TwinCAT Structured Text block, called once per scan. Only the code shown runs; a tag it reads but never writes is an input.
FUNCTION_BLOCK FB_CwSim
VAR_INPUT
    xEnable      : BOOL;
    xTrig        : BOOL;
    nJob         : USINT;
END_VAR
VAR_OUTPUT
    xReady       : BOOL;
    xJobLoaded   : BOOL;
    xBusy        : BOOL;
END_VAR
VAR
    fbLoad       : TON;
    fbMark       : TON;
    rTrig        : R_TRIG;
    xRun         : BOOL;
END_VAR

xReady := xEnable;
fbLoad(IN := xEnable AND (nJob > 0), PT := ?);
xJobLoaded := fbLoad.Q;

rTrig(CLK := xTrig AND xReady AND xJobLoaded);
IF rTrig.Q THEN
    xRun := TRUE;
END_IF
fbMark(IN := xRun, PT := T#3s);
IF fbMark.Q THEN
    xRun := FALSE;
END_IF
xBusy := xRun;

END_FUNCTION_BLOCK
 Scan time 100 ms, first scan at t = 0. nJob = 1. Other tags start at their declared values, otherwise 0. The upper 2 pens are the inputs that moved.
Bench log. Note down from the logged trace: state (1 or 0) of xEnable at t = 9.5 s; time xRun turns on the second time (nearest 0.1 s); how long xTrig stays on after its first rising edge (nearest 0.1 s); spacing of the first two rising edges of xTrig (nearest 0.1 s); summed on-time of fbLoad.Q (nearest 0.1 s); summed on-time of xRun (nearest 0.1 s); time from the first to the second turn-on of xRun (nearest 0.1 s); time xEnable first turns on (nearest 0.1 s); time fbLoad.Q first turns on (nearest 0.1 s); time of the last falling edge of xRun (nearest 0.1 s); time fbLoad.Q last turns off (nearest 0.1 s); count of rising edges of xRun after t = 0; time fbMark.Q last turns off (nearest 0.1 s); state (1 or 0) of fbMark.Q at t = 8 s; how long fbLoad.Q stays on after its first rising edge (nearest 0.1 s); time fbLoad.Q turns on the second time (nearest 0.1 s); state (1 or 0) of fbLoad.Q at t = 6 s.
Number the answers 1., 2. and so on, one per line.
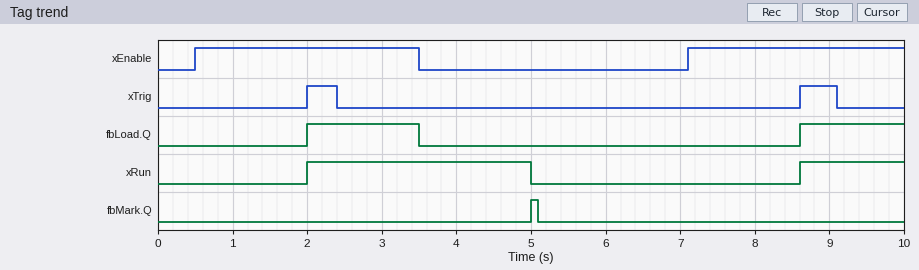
1. 1
2. 8.6 s
3. 0.4 s
4. 6.6 s
5. 2.9 s
6. 4.4 s
7. 6.6 s
8. 0.5 s
9. 2.0 s
10. 5.0 s
11. 3.5 s
12. 2
13. 5.1 s
14. 0
15. 1.5 s
16. 8.6 s
17. 0
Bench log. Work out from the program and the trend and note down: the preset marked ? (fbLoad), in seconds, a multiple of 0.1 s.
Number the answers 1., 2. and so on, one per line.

1. 1.5 s
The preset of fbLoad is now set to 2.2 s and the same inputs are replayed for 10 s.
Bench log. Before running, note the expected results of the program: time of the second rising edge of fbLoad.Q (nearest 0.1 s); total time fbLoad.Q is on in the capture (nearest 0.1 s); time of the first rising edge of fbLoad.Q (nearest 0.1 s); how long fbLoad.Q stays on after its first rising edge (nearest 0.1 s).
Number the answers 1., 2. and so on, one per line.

1. 9.3 s
2. 1.5 s
3. 2.7 s
4. 0.8 s
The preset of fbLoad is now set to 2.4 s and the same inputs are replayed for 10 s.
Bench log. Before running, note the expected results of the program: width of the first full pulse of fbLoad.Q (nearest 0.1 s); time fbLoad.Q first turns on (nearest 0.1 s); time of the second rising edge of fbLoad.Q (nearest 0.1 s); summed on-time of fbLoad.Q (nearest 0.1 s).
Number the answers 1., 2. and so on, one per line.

1. 0.6 s
2. 2.9 s
3. 9.5 s
4. 1.1 s
